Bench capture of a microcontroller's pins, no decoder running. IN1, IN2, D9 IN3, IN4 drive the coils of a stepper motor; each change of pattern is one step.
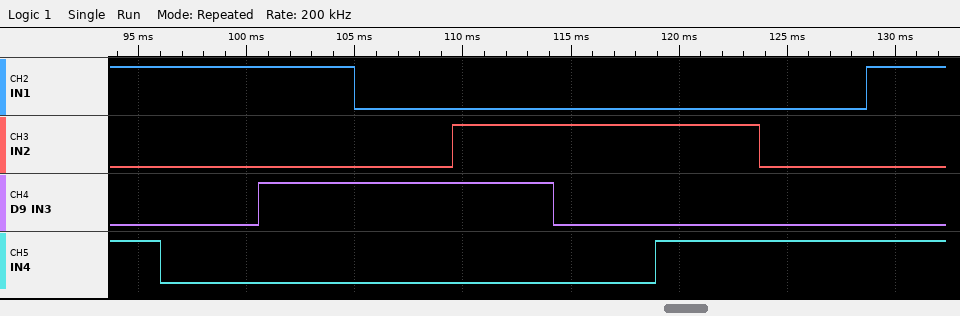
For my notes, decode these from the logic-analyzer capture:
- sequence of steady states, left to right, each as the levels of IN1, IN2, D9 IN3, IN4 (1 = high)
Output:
1001 1000 1010 0010 0110 0100 0101 0001 1001
